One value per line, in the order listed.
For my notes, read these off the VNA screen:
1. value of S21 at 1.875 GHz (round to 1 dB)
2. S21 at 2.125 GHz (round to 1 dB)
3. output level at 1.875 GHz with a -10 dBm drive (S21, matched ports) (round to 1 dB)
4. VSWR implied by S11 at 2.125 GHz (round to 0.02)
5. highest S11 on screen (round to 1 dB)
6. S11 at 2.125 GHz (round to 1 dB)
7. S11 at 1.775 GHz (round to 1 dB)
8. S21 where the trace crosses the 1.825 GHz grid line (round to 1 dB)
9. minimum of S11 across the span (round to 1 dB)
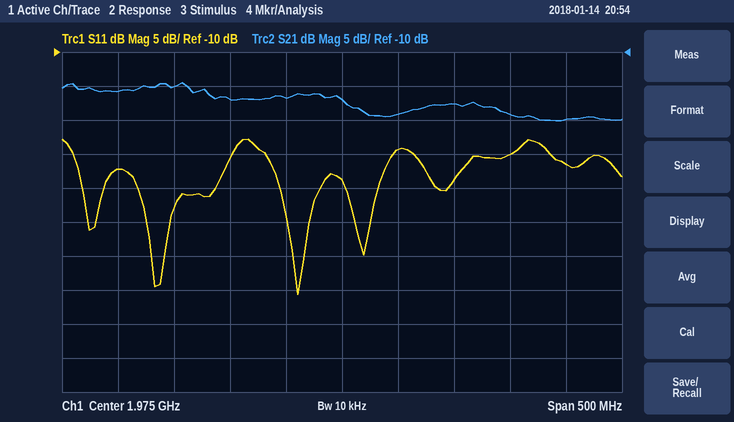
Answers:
-17 dB
-19 dB
-27 dBm
1.12
-23 dB
-25 dB
-27 dB
-15 dB
-46 dB
